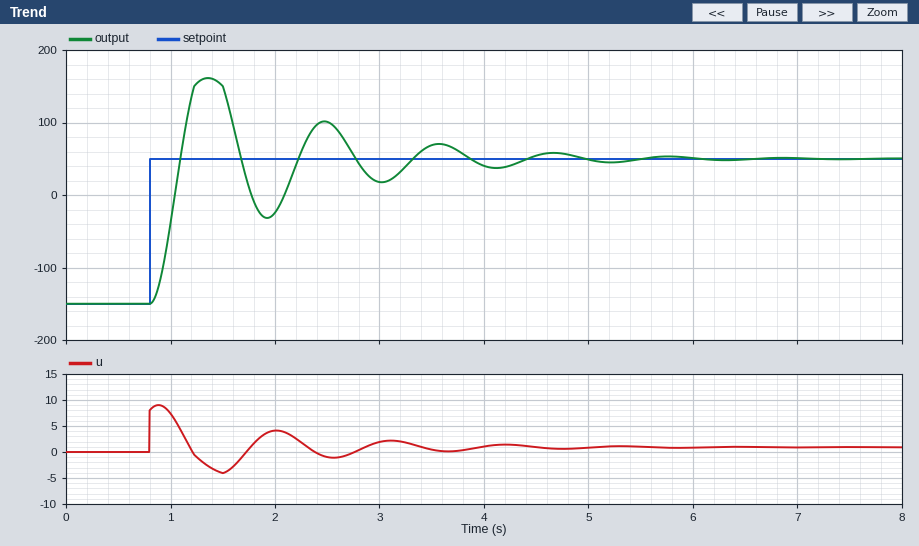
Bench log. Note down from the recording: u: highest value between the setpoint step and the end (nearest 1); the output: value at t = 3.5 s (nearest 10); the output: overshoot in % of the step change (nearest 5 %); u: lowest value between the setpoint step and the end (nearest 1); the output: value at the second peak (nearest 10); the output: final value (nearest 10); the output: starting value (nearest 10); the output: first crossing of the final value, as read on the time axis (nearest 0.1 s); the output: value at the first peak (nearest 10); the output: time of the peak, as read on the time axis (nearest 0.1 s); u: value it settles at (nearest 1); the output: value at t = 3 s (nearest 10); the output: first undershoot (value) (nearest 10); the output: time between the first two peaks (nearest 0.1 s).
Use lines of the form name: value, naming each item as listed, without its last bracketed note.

u: highest value between the setpoint step and the end: 9
the output: value at t = 3.5 s: 70
the output: overshoot in % of the step change: 55 %
u: lowest value between the setpoint step and the end: -4
the output: value at the second peak: 100
the output: final value: 50
the output: starting value: -150
the output: first crossing of the final value, as read on the time axis: 1.1 s
the output: value at the first peak: 160
the output: time of the peak, as read on the time axis: 1.4 s
u: value it settles at: 1
the output: value at t = 3 s: 20
the output: first undershoot (value): -30
the output: time between the first two peaks: 1.1 s
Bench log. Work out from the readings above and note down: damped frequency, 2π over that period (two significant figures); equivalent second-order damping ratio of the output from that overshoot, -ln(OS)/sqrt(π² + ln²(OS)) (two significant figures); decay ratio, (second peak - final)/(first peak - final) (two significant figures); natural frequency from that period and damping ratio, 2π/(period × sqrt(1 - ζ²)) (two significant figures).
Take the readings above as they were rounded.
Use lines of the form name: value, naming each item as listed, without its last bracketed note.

damped frequency, 2π over that period: 5.7 rad/s
equivalent second-order damping ratio of the output from that overshoot, -ln(OS)/sqrt(π² + ln²(OS)): 0.19
decay ratio, (second peak - final)/(first peak - final): 0.45
natural frequency from that period and damping ratio, 2π/(period × sqrt(1 - ζ²)): 5.8 rad/s
